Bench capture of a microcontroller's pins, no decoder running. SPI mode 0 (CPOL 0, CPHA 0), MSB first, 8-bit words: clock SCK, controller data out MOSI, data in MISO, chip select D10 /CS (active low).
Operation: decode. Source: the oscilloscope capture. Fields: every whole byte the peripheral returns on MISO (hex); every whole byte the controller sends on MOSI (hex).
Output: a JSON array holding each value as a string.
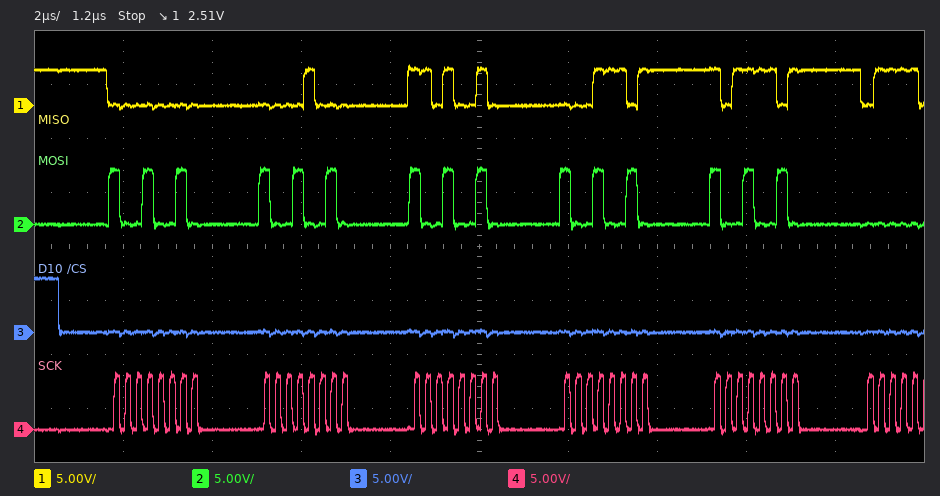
["0x00 0x08 0xD2 0x1D 0xBD", "0x92 0x92 0x92 0x92 0x92"]
